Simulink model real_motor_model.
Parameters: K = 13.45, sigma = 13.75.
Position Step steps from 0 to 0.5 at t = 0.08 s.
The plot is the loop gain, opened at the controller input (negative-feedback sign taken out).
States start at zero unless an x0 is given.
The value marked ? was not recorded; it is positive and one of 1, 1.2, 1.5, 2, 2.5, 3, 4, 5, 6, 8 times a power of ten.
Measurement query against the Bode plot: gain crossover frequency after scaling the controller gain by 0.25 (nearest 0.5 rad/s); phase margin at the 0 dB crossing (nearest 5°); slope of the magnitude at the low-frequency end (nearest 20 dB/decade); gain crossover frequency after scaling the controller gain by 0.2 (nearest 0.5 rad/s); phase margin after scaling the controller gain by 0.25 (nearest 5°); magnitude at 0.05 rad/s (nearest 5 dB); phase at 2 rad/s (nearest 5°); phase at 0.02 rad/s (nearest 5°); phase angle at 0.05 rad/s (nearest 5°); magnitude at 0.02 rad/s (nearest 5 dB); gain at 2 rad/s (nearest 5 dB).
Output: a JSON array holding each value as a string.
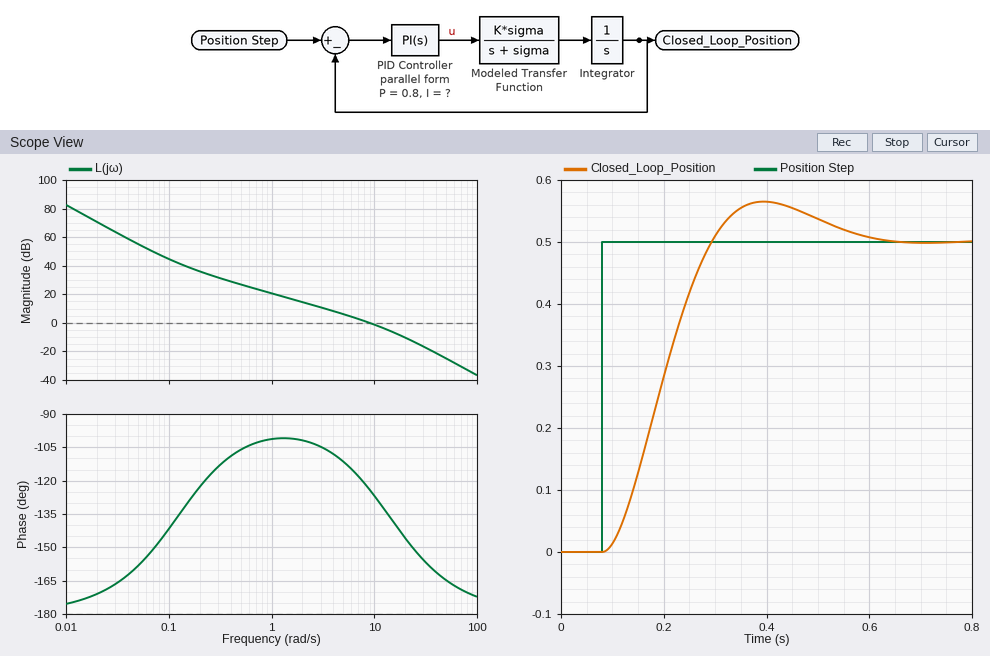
["2.5 rad/s", "55°", "-40 dB/decade", "2.0 rad/s", "75°", "55 dB", "-100°", "-170°", "-160°", "70 dB", "15 dB"]
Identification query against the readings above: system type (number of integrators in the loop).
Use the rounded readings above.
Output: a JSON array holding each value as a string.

["2"]
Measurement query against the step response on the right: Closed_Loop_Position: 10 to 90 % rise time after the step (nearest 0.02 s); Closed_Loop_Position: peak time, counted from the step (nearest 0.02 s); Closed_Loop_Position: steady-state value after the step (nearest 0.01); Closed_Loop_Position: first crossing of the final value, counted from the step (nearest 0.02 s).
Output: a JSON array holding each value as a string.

["0.14 s", "0.32 s", "0.50", "0.22 s"]
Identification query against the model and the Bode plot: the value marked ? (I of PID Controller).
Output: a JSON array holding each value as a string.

["0.1"]
